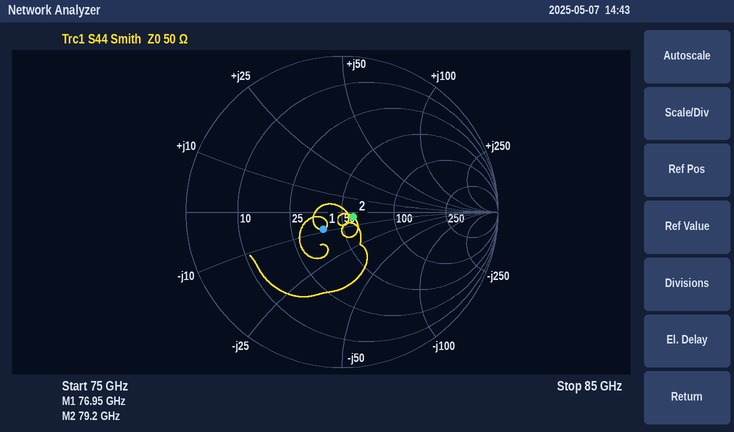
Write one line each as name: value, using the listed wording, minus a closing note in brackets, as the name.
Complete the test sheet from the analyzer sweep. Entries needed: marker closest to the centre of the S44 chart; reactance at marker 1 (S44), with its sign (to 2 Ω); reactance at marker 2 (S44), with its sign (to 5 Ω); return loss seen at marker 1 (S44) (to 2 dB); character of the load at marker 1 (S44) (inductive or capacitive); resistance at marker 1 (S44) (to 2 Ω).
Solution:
marker closest to the centre of the S44 chart: marker 2
reactance at marker 1 (S44), with its sign: -8 Ω
reactance at marker 2 (S44), with its sign: -5 Ω
return loss seen at marker 1 (S44): 16 dB
character of the load at marker 1 (S44): capacitive
resistance at marker 1 (S44): 38 Ω
